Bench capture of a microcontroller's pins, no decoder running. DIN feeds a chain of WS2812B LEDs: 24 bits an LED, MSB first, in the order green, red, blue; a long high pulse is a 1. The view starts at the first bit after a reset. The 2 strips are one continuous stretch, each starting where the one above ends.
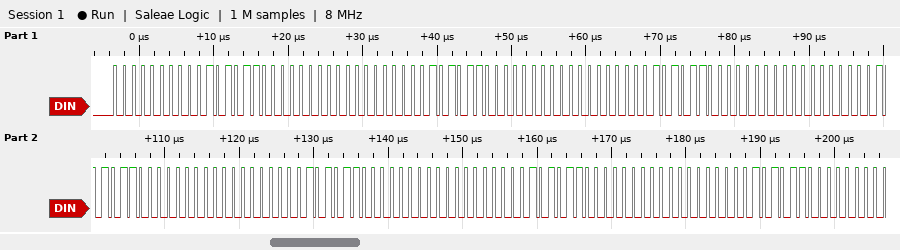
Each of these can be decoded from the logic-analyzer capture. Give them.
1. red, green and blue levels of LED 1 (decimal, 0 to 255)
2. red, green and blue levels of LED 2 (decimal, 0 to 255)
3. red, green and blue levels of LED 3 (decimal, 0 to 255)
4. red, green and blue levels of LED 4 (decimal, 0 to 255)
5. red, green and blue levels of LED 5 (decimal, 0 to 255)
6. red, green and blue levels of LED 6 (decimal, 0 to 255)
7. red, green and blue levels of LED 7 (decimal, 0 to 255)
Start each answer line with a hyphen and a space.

- 43, 0, 0
- 43, 0, 0
- 43, 0, 0
- 43, 0, 0
- 43, 0, 0
- 43, 0, 0
- 43, 0, 0
